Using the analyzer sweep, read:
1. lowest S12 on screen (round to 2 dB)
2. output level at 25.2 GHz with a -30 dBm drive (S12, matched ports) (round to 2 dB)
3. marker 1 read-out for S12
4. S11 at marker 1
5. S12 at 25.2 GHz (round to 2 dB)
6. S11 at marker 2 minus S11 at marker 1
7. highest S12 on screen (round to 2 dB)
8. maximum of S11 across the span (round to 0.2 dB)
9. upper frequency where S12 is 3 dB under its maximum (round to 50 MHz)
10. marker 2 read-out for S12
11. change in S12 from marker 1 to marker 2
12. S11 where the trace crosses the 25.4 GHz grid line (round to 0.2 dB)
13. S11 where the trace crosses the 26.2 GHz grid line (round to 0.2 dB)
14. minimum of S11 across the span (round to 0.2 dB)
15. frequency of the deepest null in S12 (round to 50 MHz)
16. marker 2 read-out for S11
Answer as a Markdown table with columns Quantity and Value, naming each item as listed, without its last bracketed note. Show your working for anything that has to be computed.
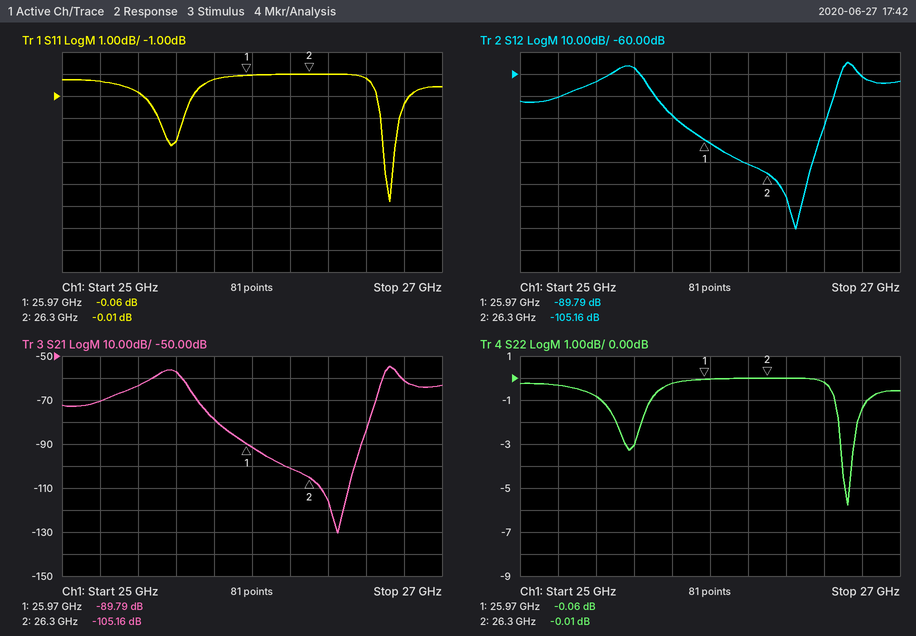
| Quantity | Value |
|---|---|
| lowest S12 on screen | -130 dB |
| output level at 25.2 GHz with a -30 dBm drive (S12, matched ports) | -30 dBm + (-70 dB) = -100 dBm |
| marker 1 read-out for S12 | -89.79 dB |
| S11 at marker 1 | -0.06 dB |
| S12 at 25.2 GHz | -70 dB |
| S11 at marker 2 minus S11 at marker 1 | -0.01 − (-0.06) = 0.05 dB |
| highest S12 on screen | -54 dB |
| maximum of S11 across the span | 0.0 dB |
| upper frequency where S12 is 3 dB under its maximum | 26.75 GHz |
| marker 2 read-out for S12 | -105.16 dB |
| change in S12 from marker 1 to marker 2 | -105.16 − (-89.79) = -15.37 dB |
| S11 where the trace crosses the 25.4 GHz grid line | -0.8 dB |
| S11 where the trace crosses the 26.2 GHz grid line | 0.0 dB |
| minimum of S11 across the span | -5.8 dB |
| frequency of the deepest null in S12 | 26.45 GHz |
| marker 2 read-out for S11 | -0.01 dB |
